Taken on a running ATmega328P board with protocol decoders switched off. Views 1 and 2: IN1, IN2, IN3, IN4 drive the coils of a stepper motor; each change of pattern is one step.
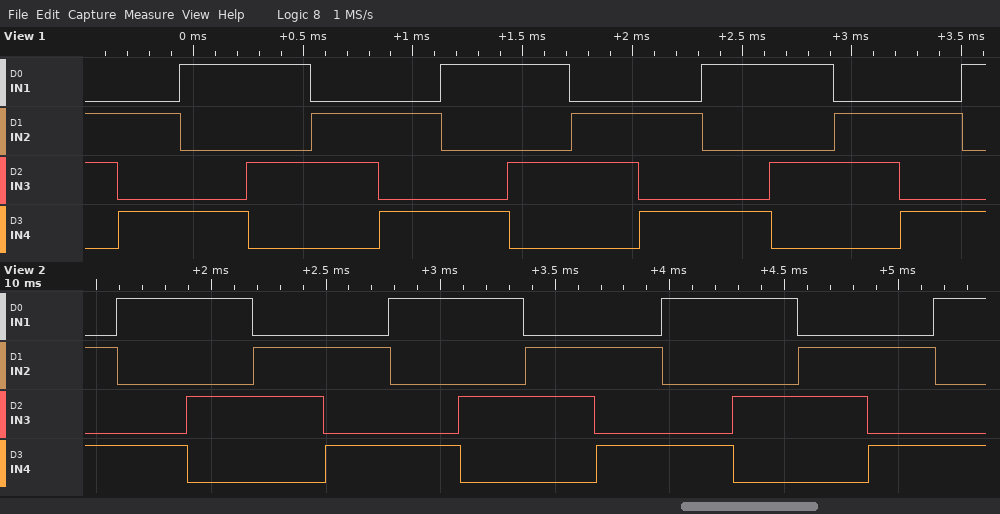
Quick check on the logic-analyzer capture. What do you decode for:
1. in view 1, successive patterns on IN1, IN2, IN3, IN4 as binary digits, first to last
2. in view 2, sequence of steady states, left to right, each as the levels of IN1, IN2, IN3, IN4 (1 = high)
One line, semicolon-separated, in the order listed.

0110 0101 1001 1010 0110 0101 1001 1010 0110 0101 1001 1010 0110 0101 1001; 0101 1001 1010 0110 0101 1001 1010 0110 0101 1001 1010 0110 0101 1001
